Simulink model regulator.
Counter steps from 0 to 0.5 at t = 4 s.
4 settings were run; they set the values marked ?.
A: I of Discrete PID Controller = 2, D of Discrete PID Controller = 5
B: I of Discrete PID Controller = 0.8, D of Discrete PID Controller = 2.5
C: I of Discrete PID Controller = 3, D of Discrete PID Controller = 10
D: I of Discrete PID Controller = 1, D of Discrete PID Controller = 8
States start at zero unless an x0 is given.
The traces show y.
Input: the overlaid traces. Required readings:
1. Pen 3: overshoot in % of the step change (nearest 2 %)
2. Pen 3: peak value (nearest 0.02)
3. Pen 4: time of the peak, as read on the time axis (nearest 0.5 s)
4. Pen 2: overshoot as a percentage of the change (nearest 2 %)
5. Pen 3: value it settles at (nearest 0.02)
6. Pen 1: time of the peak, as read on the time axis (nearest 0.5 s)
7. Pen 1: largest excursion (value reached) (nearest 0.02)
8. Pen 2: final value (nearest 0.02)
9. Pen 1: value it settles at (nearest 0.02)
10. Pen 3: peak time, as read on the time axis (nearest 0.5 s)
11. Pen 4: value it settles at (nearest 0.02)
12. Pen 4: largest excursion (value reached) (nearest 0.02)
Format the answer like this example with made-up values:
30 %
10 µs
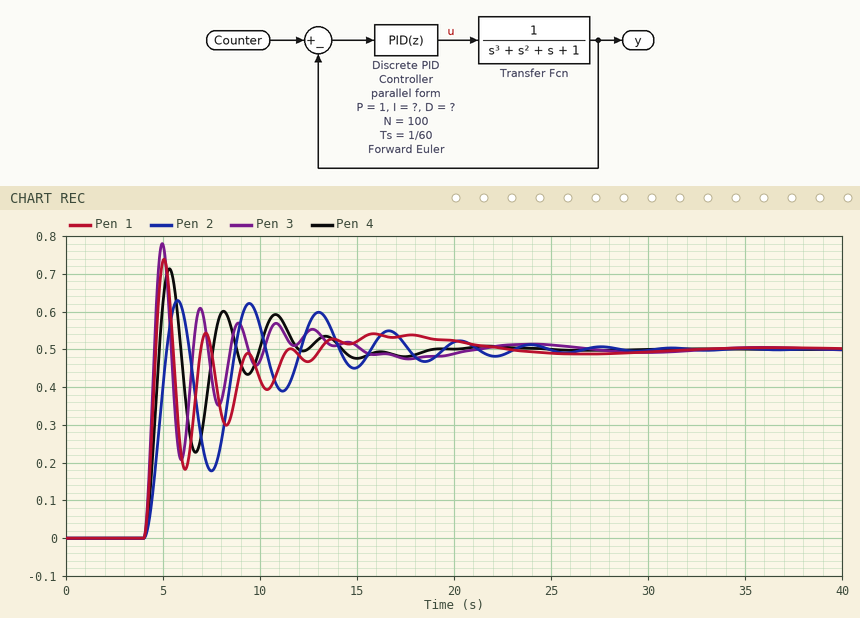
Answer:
56 %
0.78
5.5 s
26 %
0.50
5.0 s
0.74
0.50
0.50
5.0 s
0.50
0.72
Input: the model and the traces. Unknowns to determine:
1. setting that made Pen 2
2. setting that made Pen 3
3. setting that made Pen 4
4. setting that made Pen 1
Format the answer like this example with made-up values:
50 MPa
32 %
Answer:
B
C
A
D
